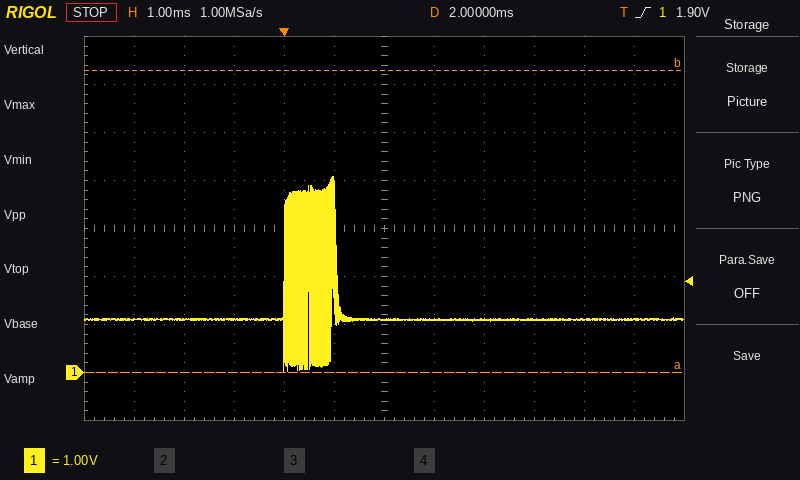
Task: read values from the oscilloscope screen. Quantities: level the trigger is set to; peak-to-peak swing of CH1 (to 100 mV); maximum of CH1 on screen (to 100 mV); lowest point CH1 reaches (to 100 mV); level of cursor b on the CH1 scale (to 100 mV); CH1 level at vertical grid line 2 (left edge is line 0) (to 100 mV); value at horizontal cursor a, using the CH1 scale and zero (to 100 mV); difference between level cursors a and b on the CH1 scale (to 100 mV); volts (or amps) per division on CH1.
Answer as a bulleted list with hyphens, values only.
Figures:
- 1.90 V
- 4.1 V
- 4.1 V
- 0.0 V
- 6.3 V
- 1.1 V
- 0.0 V
- 6.3 V
- 1 V
